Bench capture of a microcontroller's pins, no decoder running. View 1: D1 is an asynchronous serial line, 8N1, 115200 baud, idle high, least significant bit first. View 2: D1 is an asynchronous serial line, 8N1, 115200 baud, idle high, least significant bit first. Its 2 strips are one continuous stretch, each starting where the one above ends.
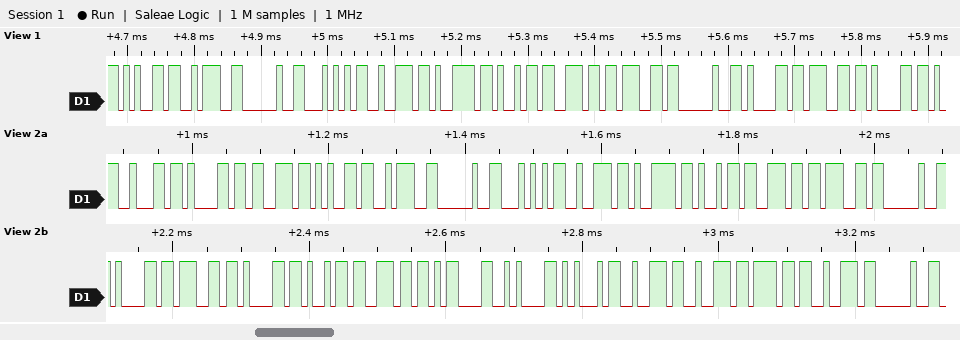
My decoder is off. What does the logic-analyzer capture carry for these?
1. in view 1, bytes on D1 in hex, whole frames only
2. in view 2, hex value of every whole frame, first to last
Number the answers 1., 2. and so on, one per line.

1. 0x65 0x3A 0x20 0x54 0x72 0x79 0x69 0x6E 0x67 0x20 0x61 0x67 0x61
2. 0x62 0x61 0x73 0x65 0x3A 0x20 0x54 0x72 0x79 0x69 0x6E 0x67 0x20 0x61 0x67 0x61 0x69 0x6E 0x0D 0x0A 0x45 0x72 0x72 0x6F 0x72 0x20
